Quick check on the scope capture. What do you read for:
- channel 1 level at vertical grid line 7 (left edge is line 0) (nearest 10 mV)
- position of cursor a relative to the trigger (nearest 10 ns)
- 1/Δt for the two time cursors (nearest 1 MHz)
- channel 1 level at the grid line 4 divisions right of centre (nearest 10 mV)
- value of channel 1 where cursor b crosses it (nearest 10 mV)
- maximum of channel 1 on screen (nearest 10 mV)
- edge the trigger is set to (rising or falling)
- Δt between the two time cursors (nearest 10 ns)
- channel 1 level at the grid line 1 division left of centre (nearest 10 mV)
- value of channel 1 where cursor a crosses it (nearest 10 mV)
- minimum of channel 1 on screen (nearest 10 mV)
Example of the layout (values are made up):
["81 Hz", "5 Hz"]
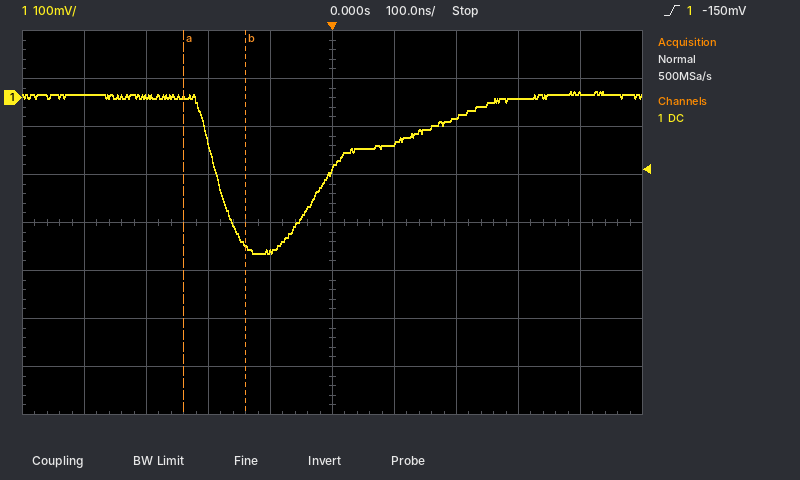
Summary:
["-40 mV", "-240 ns", "10 MHz", "10 mV", "-310 mV", "10 mV", "rising", "100 ns", "-320 mV", "0 mV", "-320 mV"]
